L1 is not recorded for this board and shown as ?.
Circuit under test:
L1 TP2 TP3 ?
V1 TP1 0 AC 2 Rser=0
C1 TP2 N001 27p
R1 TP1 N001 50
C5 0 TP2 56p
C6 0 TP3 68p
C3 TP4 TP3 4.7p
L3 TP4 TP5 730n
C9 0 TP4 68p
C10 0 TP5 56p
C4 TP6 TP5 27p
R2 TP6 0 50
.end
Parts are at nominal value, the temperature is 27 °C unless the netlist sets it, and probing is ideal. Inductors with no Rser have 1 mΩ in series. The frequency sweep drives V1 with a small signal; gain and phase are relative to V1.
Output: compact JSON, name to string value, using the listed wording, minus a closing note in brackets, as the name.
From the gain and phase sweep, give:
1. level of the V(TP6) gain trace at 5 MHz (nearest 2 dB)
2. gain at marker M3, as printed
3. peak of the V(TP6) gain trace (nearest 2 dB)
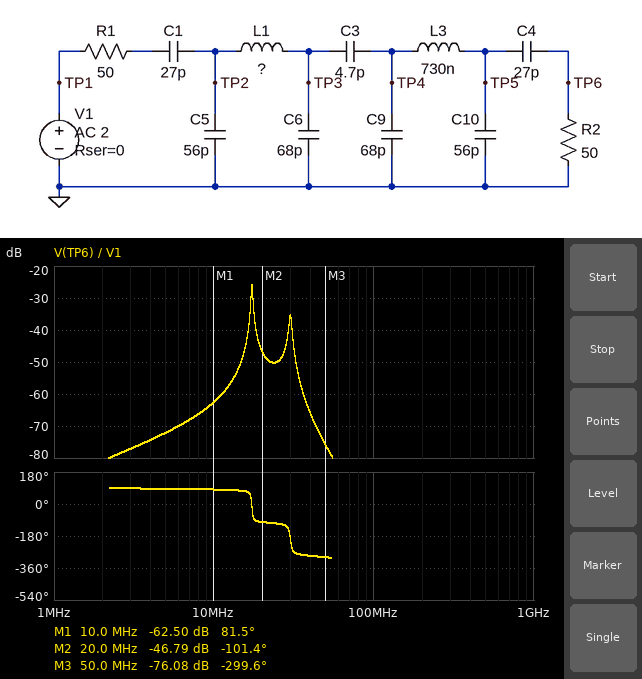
{"level of the V(TP6) gain trace at 5 MHz": "-72 dB", "gain at marker M3, as printed": "-76.08 dB", "peak of the V(TP6) gain trace": "-26 dB"}
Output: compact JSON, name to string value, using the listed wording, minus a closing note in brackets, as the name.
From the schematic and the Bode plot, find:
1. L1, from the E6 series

{"L1, from the E6 series": "2.2 µH"}
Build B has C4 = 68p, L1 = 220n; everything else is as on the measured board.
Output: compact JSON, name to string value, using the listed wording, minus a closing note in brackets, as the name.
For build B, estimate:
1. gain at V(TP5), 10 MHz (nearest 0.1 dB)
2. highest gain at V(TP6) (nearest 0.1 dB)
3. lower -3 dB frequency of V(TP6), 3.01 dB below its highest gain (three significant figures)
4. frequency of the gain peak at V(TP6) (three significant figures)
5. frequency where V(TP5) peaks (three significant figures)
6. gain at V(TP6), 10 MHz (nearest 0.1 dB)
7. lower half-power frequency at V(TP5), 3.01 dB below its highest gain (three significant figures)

{"gain at V(TP5), 10 MHz": "-46.0 dB", "highest gain at V(TP6)": "-31.0 dB", "lower -3 dB frequency of V(TP6), 3.01 dB below its highest gain": "26.5 MHz", "frequency of the gain peak at V(TP6)": "28.0 MHz", "frequency where V(TP5) peaks": "27.9 MHz", "gain at V(TP6), 10 MHz": "-59.6 dB", "lower half-power frequency at V(TP5), 3.01 dB below its highest gain": "26.4 MHz"}
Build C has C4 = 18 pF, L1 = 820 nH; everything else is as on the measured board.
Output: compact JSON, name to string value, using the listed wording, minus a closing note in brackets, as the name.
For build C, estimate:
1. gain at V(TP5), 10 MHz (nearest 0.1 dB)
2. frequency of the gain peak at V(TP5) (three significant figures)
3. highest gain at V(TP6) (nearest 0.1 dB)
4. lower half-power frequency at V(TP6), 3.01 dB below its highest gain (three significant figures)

{"gain at V(TP5), 10 MHz": "-43.0 dB", "frequency of the gain peak at V(TP5)": "30.9 MHz", "highest gain at V(TP6)": "-12.9 dB", "lower half-power frequency at V(TP6), 3.01 dB below its highest gain": "30.5 MHz"}
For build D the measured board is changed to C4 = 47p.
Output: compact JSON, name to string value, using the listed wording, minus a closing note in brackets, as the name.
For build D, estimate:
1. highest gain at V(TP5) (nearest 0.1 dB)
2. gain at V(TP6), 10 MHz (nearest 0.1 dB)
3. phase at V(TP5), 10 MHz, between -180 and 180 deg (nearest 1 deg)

{"highest gain at V(TP5)": "-9.6 dB", "gain at V(TP6), 10 MHz": "-58.7 dB", "phase at V(TP5), 10 MHz, between -180 and 180 deg": "-2 deg"}
